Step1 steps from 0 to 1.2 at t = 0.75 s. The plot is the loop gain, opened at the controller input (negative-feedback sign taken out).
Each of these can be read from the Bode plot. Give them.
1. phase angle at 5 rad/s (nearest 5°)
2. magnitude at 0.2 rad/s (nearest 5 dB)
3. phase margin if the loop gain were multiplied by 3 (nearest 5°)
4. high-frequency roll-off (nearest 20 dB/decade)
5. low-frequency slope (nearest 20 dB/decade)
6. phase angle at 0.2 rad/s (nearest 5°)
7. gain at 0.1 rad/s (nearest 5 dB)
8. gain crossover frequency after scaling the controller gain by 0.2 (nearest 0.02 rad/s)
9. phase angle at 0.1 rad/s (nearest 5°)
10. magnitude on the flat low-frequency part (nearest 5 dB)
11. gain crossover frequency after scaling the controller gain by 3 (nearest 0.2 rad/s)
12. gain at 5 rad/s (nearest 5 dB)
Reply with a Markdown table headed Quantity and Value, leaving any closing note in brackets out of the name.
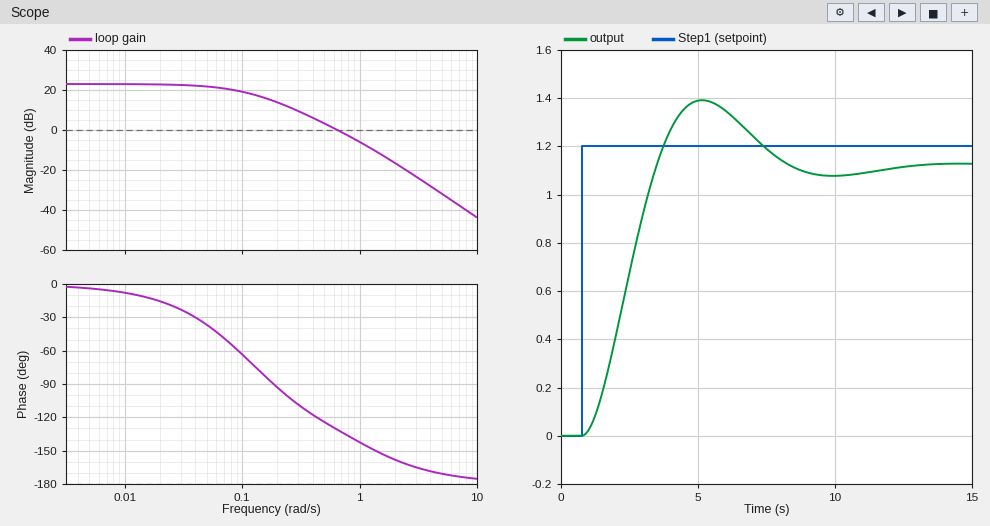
| Quantity | Value |
|---|---|
| phase angle at 5 rad/s | -170° |
| magnitude at 0.2 rad/s | 15 dB |
| phase margin if the loop gain were multiplied by 3 | 30° |
| high-frequency roll-off | -40 dB/decade |
| low-frequency slope | 0 dB/decade |
| phase angle at 0.2 rad/s | -95° |
| gain at 0.1 rad/s | 20 dB |
| gain crossover frequency after scaling the controller gain by 0.2 | 0.20 rad/s |
| phase angle at 0.1 rad/s | -65° |
| magnitude on the flat low-frequency part | 25 dB |
| gain crossover frequency after scaling the controller gain by 3 | 1.2 rad/s |
| gain at 5 rad/s | -30 dB |
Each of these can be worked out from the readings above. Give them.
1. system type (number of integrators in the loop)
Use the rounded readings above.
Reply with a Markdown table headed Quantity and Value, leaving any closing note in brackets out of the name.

| Quantity | Value |
|---|---|
| system type | 0 |
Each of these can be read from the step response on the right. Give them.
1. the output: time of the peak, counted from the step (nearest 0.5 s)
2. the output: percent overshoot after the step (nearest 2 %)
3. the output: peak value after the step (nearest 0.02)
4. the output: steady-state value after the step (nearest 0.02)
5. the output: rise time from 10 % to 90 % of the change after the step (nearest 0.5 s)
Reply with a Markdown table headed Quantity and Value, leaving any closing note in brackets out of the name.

| Quantity | Value |
|---|---|
| the output: time of the peak, counted from the step | 4.5 s |
| the output: percent overshoot after the step | 24 % |
| the output: peak value after the step | 1.40 |
| the output: steady-state value after the step | 1.12 |
| the output: rise time from 10 % to 90 % of the change after the step | 2.0 s |
